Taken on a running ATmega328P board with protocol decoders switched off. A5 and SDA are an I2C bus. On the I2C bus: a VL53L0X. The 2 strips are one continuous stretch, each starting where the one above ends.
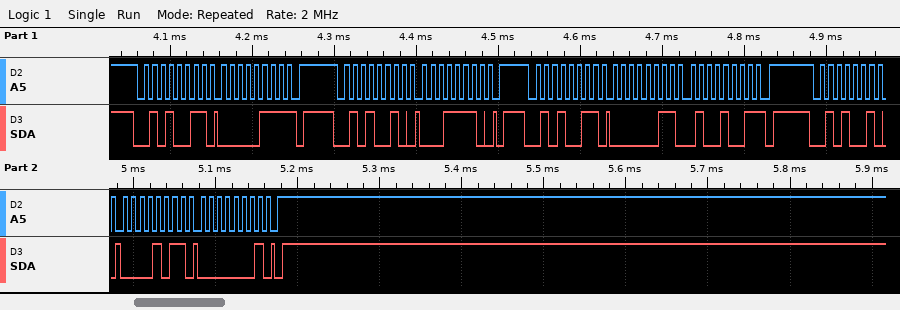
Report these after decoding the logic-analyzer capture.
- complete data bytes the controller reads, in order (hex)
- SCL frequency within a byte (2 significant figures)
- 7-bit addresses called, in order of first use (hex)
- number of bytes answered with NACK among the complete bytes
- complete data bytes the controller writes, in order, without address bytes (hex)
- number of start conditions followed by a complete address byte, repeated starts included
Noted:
07 03 49
100 kHz
0x29
2
1E 0B 01
4
